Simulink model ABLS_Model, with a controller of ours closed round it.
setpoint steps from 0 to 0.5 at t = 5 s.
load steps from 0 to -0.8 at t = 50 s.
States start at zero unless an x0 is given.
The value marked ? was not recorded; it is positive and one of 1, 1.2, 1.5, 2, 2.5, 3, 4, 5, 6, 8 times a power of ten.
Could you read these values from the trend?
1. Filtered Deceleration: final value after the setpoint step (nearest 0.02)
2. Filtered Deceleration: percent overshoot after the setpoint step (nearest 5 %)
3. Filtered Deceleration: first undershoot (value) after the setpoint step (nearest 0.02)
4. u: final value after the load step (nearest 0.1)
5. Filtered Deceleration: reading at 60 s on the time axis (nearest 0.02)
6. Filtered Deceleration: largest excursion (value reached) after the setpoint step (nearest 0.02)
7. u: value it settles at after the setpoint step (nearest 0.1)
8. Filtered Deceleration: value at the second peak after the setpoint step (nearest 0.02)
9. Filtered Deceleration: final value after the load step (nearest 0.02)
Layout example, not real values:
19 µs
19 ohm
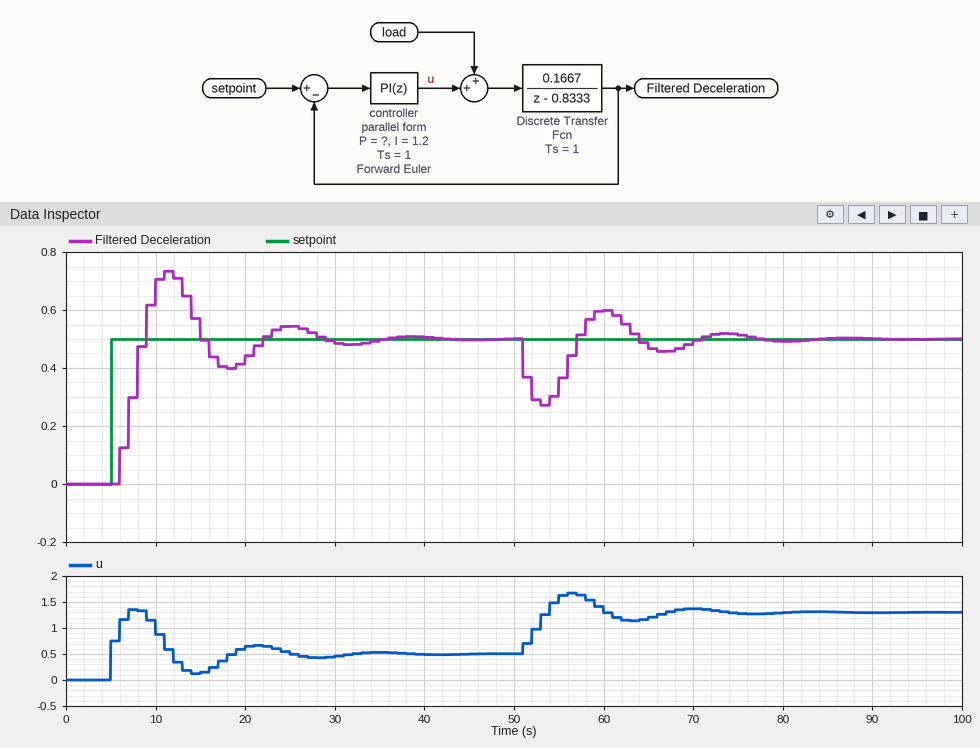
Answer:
0.50
45 %
0.40
1.3
0.60
0.74
0.5
0.54
0.50
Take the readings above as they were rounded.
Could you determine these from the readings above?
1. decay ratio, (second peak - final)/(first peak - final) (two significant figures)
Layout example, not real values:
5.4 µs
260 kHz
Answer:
0.17
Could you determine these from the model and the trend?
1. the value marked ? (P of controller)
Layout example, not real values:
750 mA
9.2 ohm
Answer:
1.5
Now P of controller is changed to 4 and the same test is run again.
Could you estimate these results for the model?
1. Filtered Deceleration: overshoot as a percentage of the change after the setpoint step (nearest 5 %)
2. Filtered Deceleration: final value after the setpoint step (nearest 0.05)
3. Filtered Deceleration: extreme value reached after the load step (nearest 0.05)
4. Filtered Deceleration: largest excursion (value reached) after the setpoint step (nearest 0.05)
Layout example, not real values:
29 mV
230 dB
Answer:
10 %
0.50
0.35
0.55
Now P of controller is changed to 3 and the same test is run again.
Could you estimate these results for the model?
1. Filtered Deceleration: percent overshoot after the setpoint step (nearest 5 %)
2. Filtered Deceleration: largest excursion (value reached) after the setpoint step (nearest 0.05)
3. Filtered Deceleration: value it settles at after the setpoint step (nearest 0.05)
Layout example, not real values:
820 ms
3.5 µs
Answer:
20 %
0.60
0.50
